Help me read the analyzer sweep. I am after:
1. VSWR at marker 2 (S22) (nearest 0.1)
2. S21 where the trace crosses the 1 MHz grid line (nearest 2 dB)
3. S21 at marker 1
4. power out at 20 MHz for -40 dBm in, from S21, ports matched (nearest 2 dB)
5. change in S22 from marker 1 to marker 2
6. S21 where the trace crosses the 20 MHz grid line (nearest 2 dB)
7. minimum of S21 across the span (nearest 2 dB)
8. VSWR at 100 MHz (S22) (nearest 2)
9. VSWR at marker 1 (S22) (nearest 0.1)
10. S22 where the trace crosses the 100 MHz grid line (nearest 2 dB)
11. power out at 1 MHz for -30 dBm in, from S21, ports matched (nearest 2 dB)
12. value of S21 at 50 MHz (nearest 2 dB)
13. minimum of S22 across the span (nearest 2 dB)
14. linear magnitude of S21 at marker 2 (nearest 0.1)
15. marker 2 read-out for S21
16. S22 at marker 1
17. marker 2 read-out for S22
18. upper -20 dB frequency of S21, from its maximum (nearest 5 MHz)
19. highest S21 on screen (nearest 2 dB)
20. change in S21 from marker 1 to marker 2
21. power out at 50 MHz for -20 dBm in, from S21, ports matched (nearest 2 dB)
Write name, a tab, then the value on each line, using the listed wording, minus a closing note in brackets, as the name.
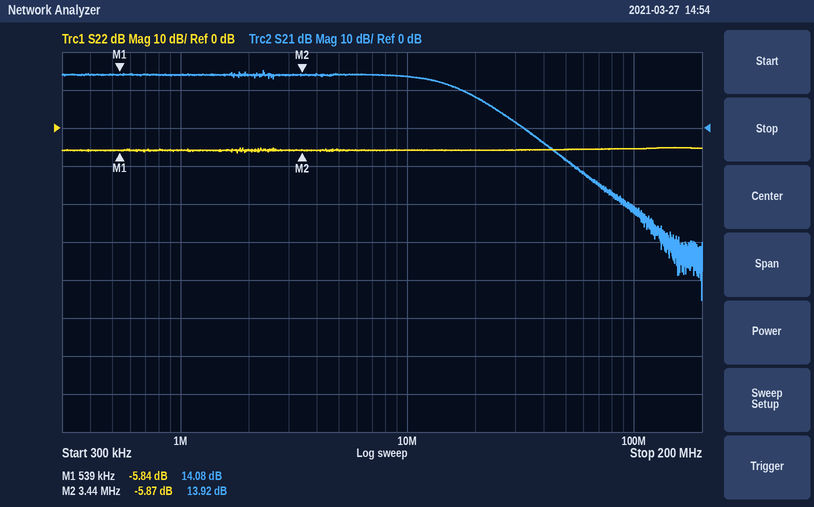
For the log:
VSWR at marker 2 (S22)	3.1
S21 where the trace crosses the 1 MHz grid line	14 dB
S21 at marker 1	14.08 dB
power out at 20 MHz for -40 dBm in, from S21, ports matched	-32 dBm
change in S22 from marker 1 to marker 2	-0.03 dB
S21 where the trace crosses the 20 MHz grid line	8 dB
minimum of S21 across the span	-46 dB
VSWR at 100 MHz (S22)	4
VSWR at marker 1 (S22)	3.1
S22 where the trace crosses the 100 MHz grid line	-6 dB
power out at 1 MHz for -30 dBm in, from S21, ports matched	-16 dBm
value of S21 at 50 MHz	-8 dB
minimum of S22 across the span	-6 dB
linear magnitude of S21 at marker 2	5.0
marker 2 read-out for S21	13.92 dB
S22 at marker 1	-5.84 dB
marker 2 read-out for S22	-5.87 dB
upper -20 dB frequency of S21, from its maximum	40 MHz
highest S21 on screen	16 dB
change in S21 from marker 1 to marker 2	-0.16 dB
power out at 50 MHz for -20 dBm in, from S21, ports matched	-28 dBm
